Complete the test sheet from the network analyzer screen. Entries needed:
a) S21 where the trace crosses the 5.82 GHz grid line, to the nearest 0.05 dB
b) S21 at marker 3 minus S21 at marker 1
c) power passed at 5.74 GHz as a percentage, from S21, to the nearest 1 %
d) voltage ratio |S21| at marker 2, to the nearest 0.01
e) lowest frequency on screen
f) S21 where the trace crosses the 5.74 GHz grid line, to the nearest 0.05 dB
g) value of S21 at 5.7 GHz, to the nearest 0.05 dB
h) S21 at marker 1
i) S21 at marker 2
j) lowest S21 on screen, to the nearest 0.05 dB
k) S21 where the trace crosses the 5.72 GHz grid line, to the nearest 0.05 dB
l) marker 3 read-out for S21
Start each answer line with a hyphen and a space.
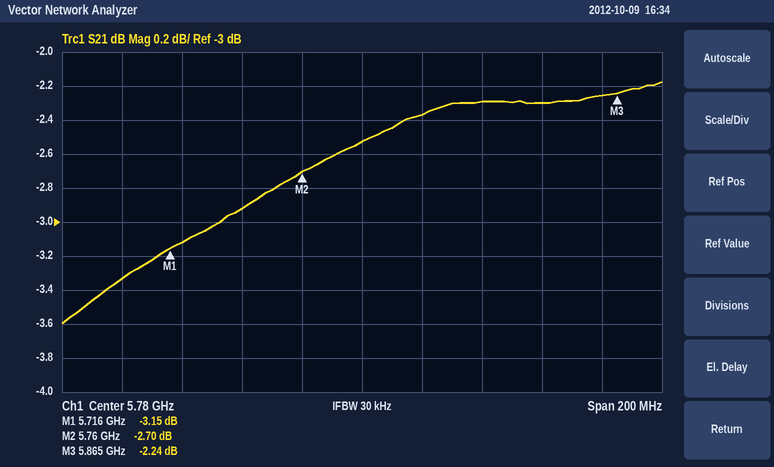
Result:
- -2.30 dB
- 0.91 dB
- 51 %
- 0.73
- 5.68 GHz
- -2.90 dB
- -3.35 dB
- -3.15 dB
- -2.70 dB
- -3.60 dB
- -3.10 dB
- -2.24 dB
